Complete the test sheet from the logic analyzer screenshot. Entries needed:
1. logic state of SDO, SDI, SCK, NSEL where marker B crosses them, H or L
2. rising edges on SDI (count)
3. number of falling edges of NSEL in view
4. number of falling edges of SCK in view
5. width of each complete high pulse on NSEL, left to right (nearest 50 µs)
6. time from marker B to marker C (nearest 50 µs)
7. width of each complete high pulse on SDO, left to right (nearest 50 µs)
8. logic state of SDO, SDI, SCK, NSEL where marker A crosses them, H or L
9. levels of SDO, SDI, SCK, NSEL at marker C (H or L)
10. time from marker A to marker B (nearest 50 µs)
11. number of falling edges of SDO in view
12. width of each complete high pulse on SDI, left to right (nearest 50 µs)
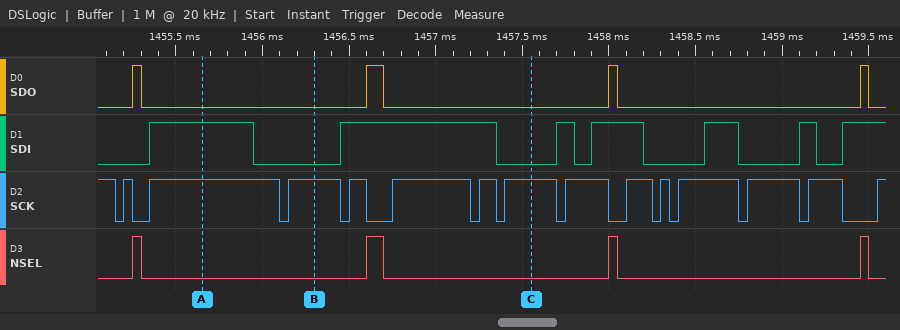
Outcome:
SDO=L, SDI=L, SCK=H, NSEL=L
7
4
14
50 µs, 100 µs, 50 µs, 50 µs
1250 µs
50 µs, 100 µs, 50 µs, 50 µs
SDO=L, SDI=H, SCK=H, NSEL=L
SDO=L, SDI=L, SCK=H, NSEL=L
650 µs
4
600 µs, 900 µs, 100 µs, 300 µs, 200 µs, 100 µs
